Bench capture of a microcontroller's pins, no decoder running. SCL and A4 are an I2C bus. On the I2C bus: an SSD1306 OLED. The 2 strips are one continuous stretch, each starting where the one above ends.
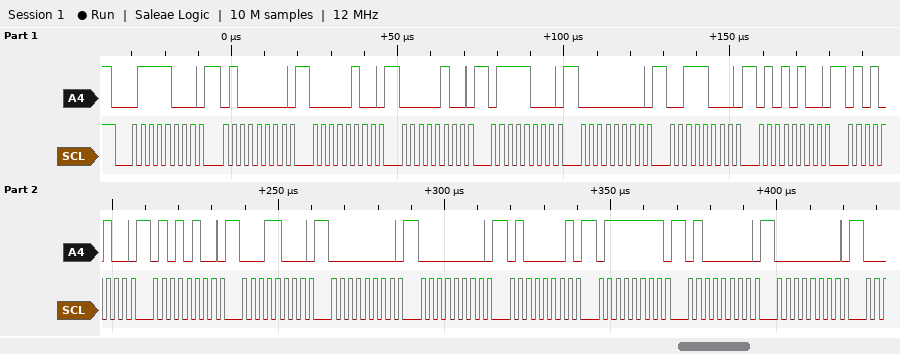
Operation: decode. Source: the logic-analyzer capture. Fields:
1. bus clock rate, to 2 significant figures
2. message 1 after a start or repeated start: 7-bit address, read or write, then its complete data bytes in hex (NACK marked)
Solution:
400 kHz
0x3C write: 40 04 04 78 00 38 54 54 54 18 00 00 41 7F 40 00
